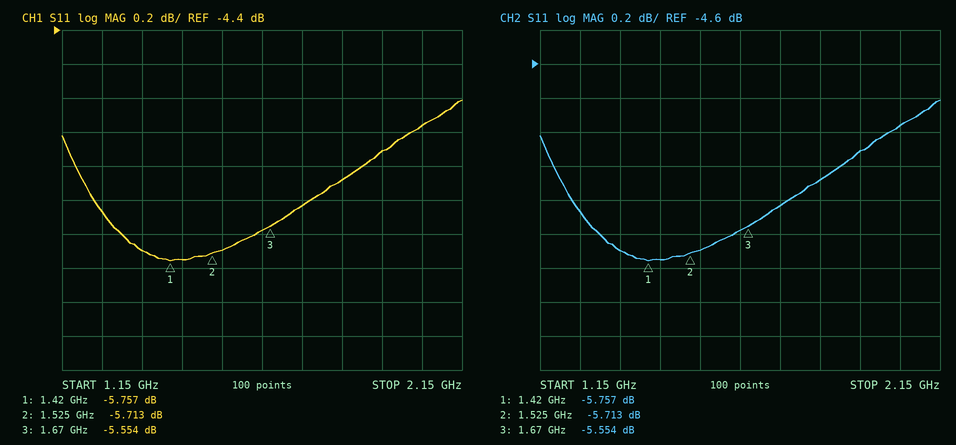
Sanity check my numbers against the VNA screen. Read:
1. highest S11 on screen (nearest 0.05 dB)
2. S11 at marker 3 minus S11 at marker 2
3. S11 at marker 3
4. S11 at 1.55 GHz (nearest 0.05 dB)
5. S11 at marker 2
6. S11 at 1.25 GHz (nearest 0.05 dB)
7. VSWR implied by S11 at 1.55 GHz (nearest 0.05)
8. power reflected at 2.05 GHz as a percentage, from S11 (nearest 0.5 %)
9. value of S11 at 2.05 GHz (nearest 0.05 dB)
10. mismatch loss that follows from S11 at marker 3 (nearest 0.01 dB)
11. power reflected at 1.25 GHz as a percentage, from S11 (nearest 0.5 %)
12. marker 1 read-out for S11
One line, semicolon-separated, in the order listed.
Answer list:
-4.80 dB; 0.159 dB; -5.554 dB; -5.70 dB; -5.713 dB; -5.45 dB; 3.15; 32.0 %; -4.95 dB; 1.42 dB; 28.5 %; -5.757 dB
